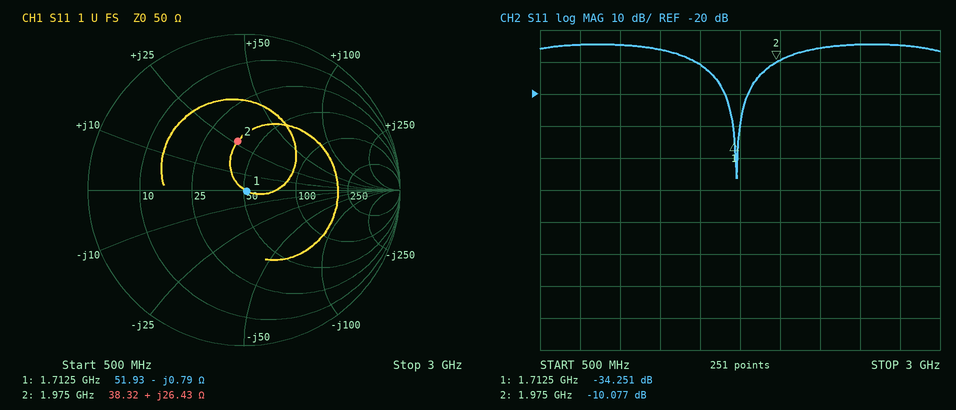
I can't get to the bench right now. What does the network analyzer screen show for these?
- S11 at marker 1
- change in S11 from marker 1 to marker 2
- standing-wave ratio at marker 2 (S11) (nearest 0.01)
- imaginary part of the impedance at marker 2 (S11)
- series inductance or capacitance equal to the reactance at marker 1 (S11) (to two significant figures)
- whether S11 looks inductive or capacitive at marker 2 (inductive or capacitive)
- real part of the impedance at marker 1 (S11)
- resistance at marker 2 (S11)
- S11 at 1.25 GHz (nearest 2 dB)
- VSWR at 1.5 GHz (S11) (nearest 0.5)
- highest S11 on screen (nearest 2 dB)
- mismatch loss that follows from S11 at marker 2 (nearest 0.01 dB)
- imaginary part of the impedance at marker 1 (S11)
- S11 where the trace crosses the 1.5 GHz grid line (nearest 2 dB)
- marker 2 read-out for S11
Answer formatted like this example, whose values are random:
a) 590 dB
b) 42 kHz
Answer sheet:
a) -34.251 dB
b) 24.174 dB
c) 1.91
d) +26.43 Ω
e) 120 pF
f) inductive
g) 51.93 Ω
h) 38.32 Ω
i) -6 dB
j) 2.0
k) -4 dB
l) 0.45 dB
m) -0.79 Ω
n) -10 dB
o) -10.077 dB
